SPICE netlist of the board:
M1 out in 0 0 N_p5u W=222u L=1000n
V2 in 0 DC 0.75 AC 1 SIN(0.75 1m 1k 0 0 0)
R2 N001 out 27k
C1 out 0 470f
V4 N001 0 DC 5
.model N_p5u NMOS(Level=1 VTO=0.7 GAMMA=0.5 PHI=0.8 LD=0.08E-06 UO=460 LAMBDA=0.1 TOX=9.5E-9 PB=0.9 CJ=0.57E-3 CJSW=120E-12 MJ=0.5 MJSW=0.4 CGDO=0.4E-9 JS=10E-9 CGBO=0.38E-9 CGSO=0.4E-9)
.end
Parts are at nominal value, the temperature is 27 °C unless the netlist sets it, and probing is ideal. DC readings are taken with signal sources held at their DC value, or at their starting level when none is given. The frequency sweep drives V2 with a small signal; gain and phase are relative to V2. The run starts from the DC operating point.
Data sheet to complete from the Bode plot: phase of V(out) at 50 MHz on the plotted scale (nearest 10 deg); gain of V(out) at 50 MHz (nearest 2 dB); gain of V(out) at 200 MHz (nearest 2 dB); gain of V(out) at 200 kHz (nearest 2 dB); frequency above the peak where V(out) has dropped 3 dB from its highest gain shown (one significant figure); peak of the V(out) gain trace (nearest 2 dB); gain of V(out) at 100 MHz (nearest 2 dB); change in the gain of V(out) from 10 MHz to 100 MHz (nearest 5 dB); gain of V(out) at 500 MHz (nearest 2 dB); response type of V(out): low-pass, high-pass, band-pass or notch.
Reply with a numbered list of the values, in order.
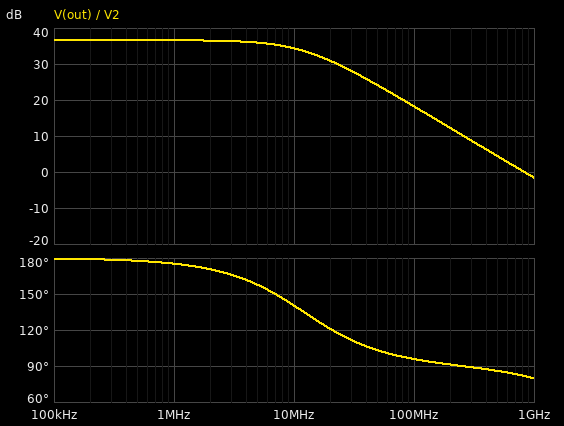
1. 100 deg
2. 24 dB
3. 12 dB
4. 36 dB
5. 10 MHz
6. 36 dB
7. 18 dB
8. -15 dB
9. 4 dB
10. low-pass
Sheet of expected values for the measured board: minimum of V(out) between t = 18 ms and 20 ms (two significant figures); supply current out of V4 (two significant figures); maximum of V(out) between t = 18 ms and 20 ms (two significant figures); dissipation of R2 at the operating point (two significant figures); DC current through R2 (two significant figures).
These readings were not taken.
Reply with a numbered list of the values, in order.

1. 3.0 V
2. 72 µA
3. 3.1 V
4. 140 µW
5. 72 µA
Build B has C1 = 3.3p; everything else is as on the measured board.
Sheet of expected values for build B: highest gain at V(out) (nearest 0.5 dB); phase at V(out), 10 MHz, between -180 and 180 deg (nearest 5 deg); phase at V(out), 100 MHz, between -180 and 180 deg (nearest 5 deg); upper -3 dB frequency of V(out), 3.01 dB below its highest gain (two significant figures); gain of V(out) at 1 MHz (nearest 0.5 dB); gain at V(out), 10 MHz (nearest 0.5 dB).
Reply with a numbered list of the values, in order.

1. 36.5 dB
2. 100 deg
3. 90 deg
4. 2.0 MHz
5. 35.5 dB
6. 22.5 dB
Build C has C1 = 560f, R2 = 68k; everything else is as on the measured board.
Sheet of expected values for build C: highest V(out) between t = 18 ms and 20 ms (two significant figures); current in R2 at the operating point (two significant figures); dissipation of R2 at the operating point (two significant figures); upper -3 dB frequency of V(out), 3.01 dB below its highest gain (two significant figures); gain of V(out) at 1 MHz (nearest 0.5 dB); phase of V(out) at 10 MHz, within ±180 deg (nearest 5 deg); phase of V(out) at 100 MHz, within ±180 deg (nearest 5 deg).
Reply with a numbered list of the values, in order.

1. 1.0 V
2. 60 µA
3. 250 µW
4. 5.0 MHz
5. 41.5 dB
6. 115 deg
7. 90 deg
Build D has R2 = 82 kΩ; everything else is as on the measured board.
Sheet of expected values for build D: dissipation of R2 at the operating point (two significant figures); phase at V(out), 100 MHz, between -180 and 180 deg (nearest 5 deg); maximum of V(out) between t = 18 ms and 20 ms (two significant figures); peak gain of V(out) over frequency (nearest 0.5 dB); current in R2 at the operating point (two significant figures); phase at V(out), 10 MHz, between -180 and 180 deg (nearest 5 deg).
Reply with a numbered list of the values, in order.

1. 270 µW
2. 90 deg
3. 450 mV
4. 42.0 dB
5. 57 µA
6. 115 deg
